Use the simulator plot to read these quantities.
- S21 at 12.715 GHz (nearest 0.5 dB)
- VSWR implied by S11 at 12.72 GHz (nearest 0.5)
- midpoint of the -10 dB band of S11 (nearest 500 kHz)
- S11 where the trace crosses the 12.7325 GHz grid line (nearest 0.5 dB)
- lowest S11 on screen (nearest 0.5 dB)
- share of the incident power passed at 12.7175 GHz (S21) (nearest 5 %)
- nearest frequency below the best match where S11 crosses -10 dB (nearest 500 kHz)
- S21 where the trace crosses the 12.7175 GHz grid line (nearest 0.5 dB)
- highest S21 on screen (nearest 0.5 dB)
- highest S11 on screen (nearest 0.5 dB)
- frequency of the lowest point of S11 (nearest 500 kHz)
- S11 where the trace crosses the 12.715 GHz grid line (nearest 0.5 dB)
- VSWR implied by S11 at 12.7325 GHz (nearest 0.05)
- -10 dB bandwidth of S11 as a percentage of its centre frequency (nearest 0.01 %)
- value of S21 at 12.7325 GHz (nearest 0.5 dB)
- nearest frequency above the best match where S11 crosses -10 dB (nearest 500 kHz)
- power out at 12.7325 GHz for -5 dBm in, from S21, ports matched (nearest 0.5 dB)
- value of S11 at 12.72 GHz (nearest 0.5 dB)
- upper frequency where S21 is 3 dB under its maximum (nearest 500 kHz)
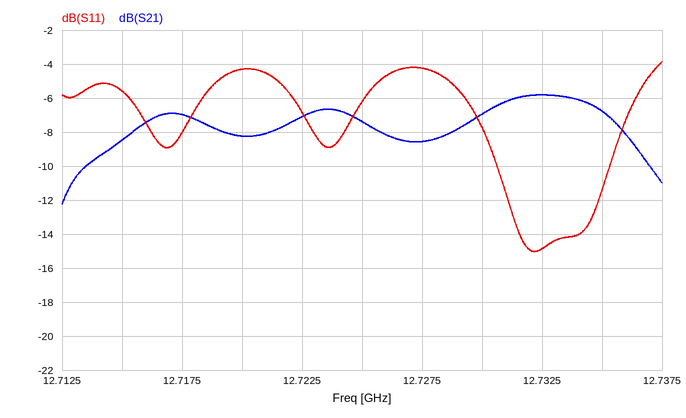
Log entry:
-8.5 dB
4.0
12.7330 GHz
-15.0 dB
-15.0 dB
20 %
12.7305 GHz
-7.0 dB
-6.0 dB
-4.0 dB
12.7320 GHz
-5.5 dB
1.45
0.04 %
-6.0 dB
12.7355 GHz
-11.0 dBm
-4.5 dB
12.7365 GHz
